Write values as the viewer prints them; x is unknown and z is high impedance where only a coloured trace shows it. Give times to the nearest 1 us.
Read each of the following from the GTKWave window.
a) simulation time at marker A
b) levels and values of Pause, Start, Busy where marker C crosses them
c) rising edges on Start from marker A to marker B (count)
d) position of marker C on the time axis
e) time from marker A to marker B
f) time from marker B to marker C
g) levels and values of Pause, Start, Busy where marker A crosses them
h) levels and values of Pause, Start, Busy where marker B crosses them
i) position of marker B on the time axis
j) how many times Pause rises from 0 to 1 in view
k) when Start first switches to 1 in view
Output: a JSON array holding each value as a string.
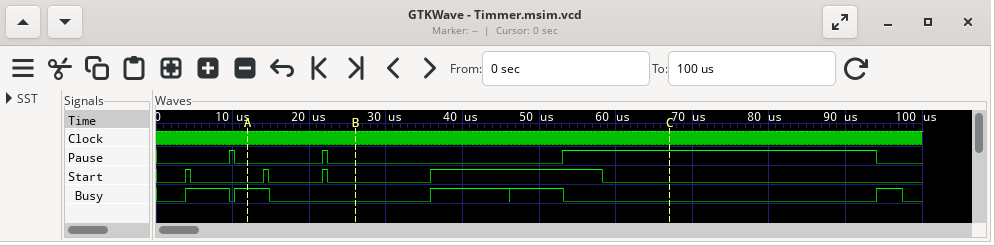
["12 us", "Pause=1, Start=0, Busy=0", "2", "67 us", "14 us", "41 us", "Pause=0, Start=0, Busy=1", "Pause=0, Start=0, Busy=0", "26 us", "3", "4 us"]
